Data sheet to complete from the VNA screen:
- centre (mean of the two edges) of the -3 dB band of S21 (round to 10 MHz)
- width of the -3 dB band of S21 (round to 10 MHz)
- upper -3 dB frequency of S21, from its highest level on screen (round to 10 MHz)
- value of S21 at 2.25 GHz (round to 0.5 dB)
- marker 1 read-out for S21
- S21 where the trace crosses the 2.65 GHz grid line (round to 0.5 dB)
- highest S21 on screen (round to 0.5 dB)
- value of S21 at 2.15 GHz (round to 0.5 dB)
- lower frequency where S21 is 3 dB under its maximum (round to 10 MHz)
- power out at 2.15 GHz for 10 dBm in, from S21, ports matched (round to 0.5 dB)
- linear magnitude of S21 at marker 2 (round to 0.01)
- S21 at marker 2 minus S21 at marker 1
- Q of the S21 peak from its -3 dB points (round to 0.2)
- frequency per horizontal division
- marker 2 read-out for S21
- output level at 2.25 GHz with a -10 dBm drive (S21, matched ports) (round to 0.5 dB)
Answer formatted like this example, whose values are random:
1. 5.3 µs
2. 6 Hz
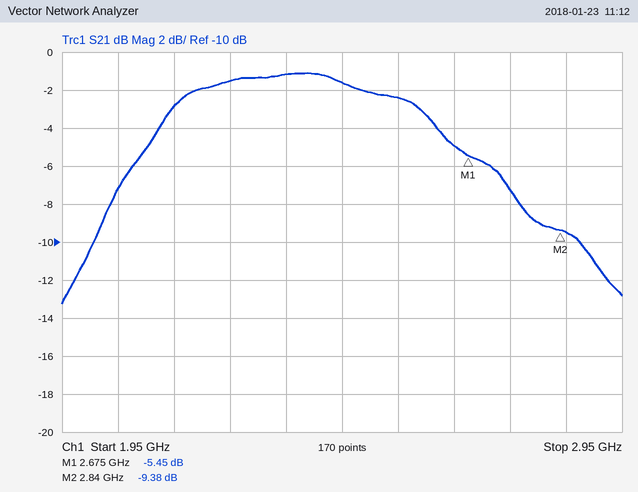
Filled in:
1. 2.37 GHz
2. 500 MHz
3. 2.62 GHz
4. -1.5 dB
5. -5.45 dB
6. -5.0 dB
7. -1.0 dB
8. -3.0 dB
9. 2.12 GHz
10. 7.0 dBm
11. 0.34
12. -3.93 dB
13. 4.8
14. 100 MHz
15. -9.38 dB
16. -11.5 dBm
